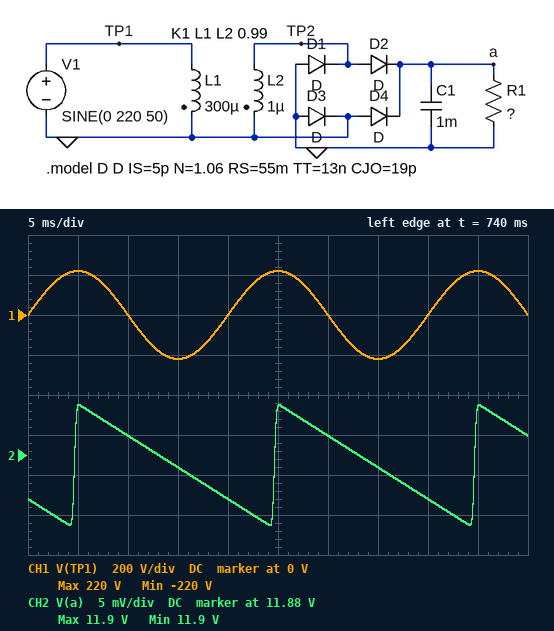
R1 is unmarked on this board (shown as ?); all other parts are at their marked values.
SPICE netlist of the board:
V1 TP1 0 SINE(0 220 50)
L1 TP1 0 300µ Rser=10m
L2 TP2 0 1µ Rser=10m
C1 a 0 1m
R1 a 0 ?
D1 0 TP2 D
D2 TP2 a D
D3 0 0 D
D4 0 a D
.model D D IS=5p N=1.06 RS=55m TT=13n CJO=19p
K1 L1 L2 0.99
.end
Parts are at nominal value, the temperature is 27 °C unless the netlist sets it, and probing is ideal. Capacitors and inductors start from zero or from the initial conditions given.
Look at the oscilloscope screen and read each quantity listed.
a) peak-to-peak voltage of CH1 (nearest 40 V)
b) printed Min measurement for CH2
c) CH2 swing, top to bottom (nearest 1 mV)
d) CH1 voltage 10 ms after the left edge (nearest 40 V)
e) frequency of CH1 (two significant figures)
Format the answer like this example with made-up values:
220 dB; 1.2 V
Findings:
440 V; 11.9 V; 15 mV; 0 V; 50 Hz
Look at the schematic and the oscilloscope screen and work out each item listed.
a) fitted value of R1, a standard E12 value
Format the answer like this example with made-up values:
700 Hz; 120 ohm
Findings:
15 kΩ
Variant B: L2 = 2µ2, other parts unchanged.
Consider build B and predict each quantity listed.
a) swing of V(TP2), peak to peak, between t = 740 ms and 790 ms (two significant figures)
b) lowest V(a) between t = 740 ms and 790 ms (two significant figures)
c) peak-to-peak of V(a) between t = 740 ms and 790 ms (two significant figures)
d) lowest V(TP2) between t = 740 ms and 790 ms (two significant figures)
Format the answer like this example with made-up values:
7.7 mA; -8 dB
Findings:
34 V; 18 V; 23 mV; -16 V
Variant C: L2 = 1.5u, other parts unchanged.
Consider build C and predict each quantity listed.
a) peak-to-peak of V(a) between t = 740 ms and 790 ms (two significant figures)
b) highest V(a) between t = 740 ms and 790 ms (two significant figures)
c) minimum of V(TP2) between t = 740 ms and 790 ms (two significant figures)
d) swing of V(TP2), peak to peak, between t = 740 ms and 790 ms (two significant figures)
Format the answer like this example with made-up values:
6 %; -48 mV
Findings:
19 mV; 15 V; -13 V; 28 V
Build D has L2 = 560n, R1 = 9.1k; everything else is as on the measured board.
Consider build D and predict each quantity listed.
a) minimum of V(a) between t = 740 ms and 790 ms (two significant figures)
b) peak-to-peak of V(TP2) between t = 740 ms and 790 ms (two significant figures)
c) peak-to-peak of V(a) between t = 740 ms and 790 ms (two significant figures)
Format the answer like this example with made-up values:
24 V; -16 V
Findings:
8.7 V; 17 V; 18 mV
